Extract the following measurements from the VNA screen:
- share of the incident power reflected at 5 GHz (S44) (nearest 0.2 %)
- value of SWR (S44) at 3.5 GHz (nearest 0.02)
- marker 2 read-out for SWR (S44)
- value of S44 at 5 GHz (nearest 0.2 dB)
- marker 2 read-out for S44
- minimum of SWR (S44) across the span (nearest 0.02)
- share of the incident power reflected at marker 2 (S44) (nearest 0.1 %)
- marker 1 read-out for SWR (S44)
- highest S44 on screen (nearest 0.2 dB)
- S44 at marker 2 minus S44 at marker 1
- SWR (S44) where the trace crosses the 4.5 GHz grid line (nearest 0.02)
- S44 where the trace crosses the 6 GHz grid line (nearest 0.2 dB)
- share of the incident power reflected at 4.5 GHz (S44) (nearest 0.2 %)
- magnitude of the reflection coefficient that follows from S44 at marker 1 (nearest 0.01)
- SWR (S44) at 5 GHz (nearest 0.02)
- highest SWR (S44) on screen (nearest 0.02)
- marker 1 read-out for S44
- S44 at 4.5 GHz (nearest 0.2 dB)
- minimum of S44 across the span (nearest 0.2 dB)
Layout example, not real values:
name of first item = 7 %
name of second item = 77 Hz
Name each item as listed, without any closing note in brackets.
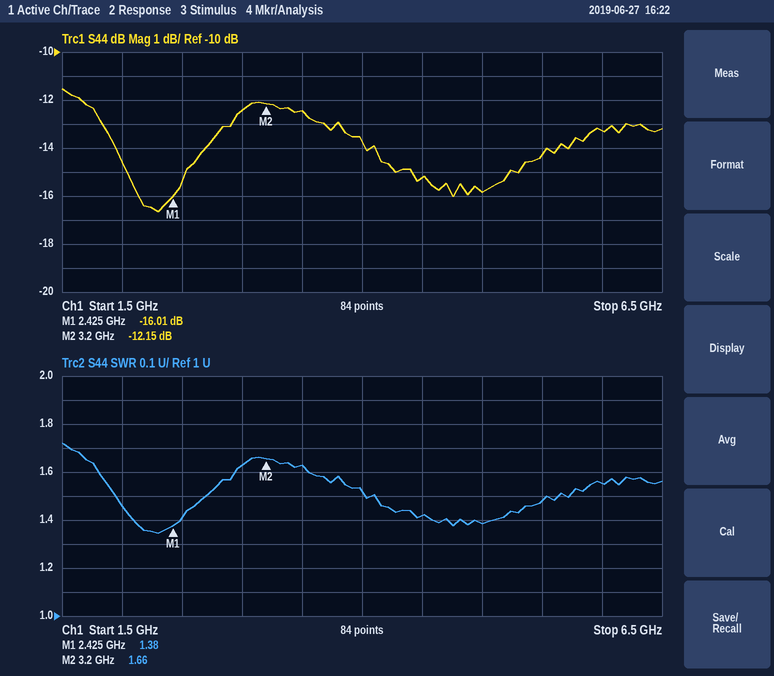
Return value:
share of the incident power reflected at 5 GHz (S44) = 2.6 %
value of SWR (S44) at 3.5 GHz = 1.62
marker 2 read-out for SWR = 1.66
value of S44 at 5 GHz = -15.8 dB
marker 2 read-out for S44 = -12.15 dB
minimum of SWR (S44) across the span = 1.34
share of the incident power reflected at marker 2 (S44) = 6.1 %
marker 1 read-out for SWR = 1.38
highest S44 on screen = -11.6 dB
S44 at marker 2 minus S44 at marker 1 = 3.86 dB
SWR (S44) where the trace crosses the 4.5 GHz grid line = 1.42
S44 where the trace crosses the 6 GHz grid line = -13.2 dB
share of the incident power reflected at 4.5 GHz (S44) = 3.0 %
magnitude of the reflection coefficient that follows from S44 at marker 1 = 0.16
SWR (S44) at 5 GHz = 1.38
highest SWR (S44) on screen = 1.72
marker 1 read-out for S44 = -16.01 dB
S44 at 4.5 GHz = -15.2 dB
minimum of S44 across the span = -16.6 dB
